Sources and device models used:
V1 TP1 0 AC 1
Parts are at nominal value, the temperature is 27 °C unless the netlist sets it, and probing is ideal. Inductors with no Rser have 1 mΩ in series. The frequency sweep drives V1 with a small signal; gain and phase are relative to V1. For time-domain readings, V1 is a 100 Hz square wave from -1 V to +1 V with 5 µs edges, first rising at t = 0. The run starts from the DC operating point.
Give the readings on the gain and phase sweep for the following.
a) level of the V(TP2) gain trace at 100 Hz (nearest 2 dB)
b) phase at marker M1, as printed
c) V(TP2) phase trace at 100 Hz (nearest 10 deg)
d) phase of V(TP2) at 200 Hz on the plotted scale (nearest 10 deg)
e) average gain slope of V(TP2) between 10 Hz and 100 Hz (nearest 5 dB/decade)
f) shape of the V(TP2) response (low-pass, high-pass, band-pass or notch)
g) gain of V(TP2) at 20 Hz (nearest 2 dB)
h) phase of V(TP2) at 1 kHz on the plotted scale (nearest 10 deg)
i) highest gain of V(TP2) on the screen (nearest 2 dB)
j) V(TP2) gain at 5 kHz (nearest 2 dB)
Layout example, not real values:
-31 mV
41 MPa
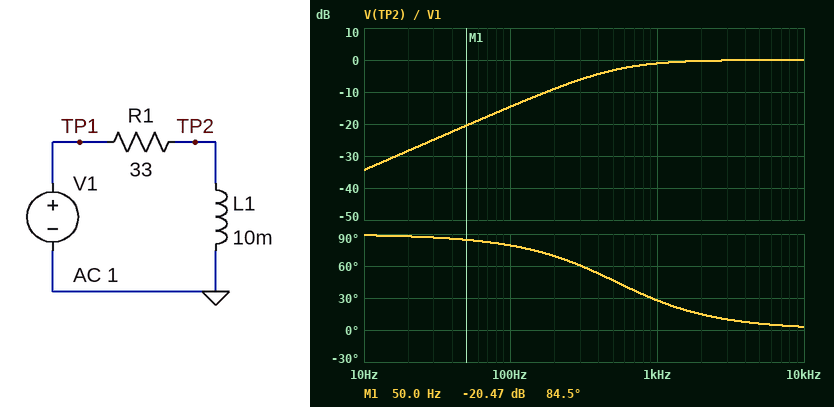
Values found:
-14 dB
84.5 deg
80 deg
70 deg
20 dB/decade
high-pass
-28 dB
30 deg
0 dB
0 dB
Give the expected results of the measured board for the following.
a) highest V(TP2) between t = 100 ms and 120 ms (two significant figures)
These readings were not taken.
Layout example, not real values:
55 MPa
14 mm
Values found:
2.0 V
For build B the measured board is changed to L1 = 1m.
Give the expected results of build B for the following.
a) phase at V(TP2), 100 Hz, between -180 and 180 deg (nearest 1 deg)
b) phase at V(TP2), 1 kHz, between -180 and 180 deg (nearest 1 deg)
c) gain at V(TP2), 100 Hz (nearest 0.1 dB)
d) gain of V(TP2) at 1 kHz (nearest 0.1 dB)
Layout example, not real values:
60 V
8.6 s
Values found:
89 deg
79 deg
-34.4 dB
-14.6 dB
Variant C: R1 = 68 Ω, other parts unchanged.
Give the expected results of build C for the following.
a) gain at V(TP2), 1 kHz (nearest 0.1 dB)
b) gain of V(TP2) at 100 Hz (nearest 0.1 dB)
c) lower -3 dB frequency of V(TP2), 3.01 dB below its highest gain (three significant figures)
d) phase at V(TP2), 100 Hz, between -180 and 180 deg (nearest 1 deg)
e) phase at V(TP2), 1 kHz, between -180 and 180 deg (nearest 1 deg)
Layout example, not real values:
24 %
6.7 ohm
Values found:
-3.4 dB
-20.7 dB
1.08 kHz
85 deg
47 deg
